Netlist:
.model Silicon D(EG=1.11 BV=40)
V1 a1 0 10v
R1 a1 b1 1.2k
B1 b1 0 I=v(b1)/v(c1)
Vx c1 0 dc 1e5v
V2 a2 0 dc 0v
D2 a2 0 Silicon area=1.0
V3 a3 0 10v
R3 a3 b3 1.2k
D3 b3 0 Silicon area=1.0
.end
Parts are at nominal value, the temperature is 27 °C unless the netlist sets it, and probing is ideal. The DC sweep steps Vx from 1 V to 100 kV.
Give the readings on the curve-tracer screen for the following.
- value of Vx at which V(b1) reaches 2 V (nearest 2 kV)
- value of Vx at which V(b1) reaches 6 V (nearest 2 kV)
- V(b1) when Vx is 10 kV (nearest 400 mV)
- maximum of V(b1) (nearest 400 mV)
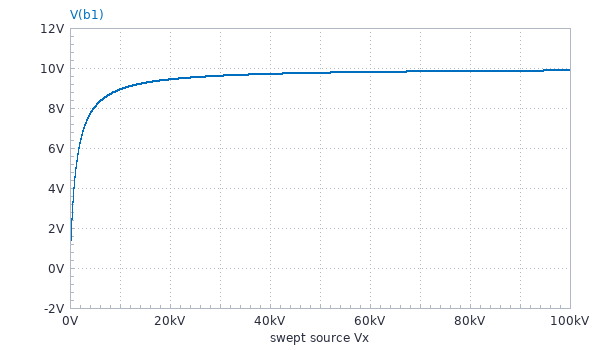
0 V
2 kV
8.8 V
10.0 V
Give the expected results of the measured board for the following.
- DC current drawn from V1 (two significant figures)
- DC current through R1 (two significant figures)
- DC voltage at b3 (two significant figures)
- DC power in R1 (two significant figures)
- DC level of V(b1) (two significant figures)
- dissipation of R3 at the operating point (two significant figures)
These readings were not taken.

99 µA
99 µA
710 mV
12 µW
9.9 V
72 mW
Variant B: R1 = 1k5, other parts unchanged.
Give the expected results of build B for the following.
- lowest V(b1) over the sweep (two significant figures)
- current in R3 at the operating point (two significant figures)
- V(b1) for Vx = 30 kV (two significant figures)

6.7 mV
7.7 mA
9.5 V
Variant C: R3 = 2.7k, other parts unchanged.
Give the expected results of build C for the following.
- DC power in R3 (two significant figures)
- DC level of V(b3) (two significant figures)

32 mW
690 mV
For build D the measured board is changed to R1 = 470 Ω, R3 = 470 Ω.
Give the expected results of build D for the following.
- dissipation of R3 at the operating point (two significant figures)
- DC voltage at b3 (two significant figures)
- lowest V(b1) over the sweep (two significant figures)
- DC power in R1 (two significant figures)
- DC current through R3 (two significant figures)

180 mW
730 mV
21 mV
4.7 µW
20 mA
